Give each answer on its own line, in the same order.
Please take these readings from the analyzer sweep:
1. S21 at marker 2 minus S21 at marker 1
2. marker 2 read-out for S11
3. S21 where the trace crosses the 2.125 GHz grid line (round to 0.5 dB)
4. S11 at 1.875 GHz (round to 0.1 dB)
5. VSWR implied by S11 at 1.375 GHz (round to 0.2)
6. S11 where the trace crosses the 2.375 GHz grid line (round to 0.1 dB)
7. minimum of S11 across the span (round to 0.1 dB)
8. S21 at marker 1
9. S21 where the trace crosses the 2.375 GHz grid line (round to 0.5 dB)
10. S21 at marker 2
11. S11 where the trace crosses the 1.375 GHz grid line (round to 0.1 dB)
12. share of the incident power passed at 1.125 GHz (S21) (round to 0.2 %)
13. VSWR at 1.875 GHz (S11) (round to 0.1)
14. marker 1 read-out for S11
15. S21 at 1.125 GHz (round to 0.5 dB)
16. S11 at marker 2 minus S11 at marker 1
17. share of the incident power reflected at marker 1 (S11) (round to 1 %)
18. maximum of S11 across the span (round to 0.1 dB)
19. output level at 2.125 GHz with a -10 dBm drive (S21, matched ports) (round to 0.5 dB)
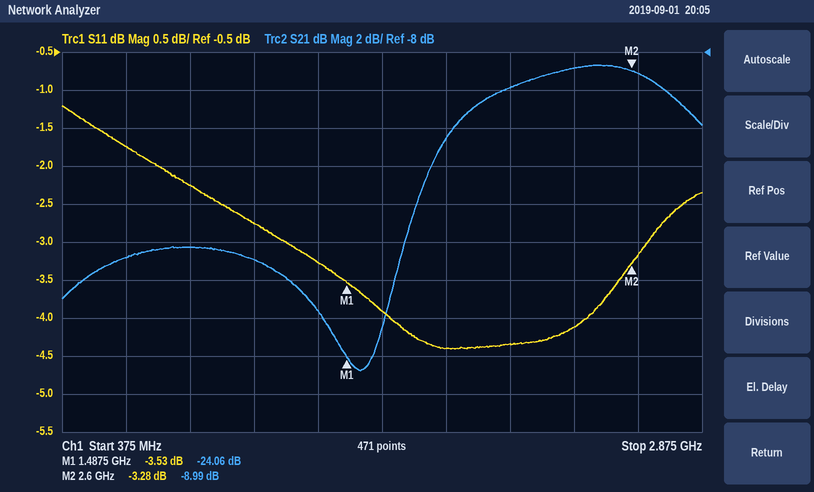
15.07 dB
-3.28 dB
-10.0 dB
-4.4 dB
5.4
-4.1 dB
-4.4 dB
-24.06 dB
-9.0 dB
-8.99 dB
-3.3 dB
1.2 %
4.0
-3.53 dB
-19.0 dB
0.25 dB
44 %
-1.2 dB
-20.0 dBm
